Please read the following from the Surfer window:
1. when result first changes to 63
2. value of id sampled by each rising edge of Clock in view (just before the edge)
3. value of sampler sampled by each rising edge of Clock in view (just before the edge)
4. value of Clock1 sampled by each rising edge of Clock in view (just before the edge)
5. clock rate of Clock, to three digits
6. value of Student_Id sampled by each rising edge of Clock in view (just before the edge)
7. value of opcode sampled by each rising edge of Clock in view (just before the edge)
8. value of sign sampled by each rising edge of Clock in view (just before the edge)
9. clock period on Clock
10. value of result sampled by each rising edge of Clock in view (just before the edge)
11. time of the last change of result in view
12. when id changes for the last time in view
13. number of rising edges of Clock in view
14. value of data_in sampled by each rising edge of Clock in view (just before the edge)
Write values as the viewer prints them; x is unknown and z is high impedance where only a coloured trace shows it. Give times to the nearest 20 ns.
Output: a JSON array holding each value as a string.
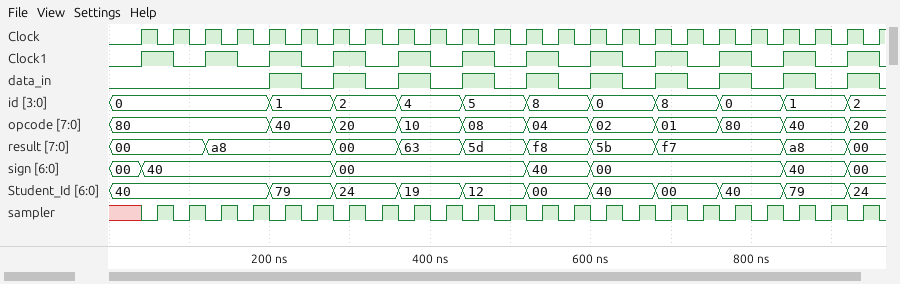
["360 ns", "0, 0, 0, 0, 0, 1, 1, 2, 2, 4, 4, 5, 5, 8, 8, 0, 0, 8, 8, 0, 0, 1, 1, 2", "x 1 1 1 1 1 1 1 1 1 1 1 1 1 1 1 1 1 1 1 1 1 1 1", "0 1 0 1 0 1 0 1 0 1 0 1 0 1 0 1 0 1 0 1 0 1 0 1", "25.0 MHz", "40, 40, 40, 40, 40, 79, 79, 24, 24, 19, 19, 12, 12, 00, 00, 40, 40, 00, 00, 40, 40, 79, 79, 24", "80, 80, 80, 80, 80, 40, 40, 20, 20, 10, 10, 08, 08, 04, 04, 02, 02, 01, 01, 80, 80, 40, 40, 20", "00, 40, 40, 40, 40, 40, 40, 00, 00, 00, 00, 00, 00, 40, 40, 00, 00, 00, 00, 00, 00, 40, 40, 00", "40 ns", "00, 00, 00, a8, a8, a8, a8, 00, 00, 63, 63, 5d, 5d, f8, f8, 5b, 5b, f7, f7, f7, f7, a8, a8, 00", "920 ns", "920 ns", "24", "0 0 0 0 0 1 0 1 0 1 0 1 0 1 0 1 0 1 0 1 0 1 0 1"]
